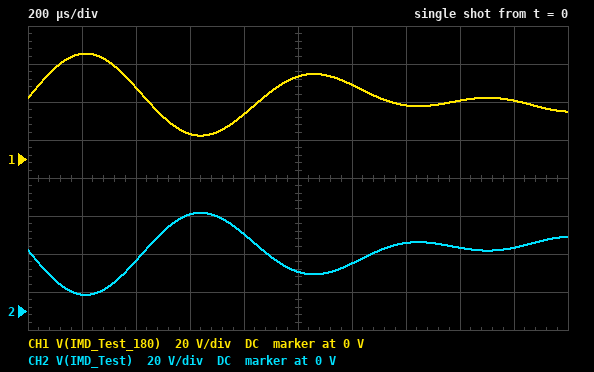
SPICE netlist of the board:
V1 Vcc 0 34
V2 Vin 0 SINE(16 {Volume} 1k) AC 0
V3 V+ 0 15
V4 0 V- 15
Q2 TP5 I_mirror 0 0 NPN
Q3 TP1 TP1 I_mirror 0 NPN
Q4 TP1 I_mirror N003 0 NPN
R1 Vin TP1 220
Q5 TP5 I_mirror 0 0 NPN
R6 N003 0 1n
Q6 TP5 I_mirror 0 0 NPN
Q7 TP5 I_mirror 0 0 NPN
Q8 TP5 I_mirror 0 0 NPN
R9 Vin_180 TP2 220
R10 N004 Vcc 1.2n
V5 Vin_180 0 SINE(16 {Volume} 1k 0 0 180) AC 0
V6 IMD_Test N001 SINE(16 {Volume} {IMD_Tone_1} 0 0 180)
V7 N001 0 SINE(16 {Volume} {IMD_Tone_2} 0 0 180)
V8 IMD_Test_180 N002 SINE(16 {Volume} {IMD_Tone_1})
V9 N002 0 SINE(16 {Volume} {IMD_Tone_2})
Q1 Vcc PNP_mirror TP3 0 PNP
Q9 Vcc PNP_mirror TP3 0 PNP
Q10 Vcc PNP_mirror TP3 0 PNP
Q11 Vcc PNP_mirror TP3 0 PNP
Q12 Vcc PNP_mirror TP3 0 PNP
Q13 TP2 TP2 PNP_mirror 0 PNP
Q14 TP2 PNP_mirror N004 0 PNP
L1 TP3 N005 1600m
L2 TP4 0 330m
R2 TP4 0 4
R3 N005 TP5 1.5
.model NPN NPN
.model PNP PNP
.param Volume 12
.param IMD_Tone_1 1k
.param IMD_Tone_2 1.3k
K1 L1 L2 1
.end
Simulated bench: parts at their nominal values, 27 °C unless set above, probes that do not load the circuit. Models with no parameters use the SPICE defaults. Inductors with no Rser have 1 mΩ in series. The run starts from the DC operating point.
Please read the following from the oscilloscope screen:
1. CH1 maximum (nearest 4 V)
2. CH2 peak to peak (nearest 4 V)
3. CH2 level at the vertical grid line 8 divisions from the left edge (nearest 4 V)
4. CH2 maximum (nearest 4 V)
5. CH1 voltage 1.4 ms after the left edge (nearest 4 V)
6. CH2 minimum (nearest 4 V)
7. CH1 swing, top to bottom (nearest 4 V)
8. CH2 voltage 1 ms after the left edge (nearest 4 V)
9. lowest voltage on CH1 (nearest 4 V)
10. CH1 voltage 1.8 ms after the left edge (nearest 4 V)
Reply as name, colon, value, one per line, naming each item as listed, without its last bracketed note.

CH1 maximum: 56 V
CH2 peak to peak: 44 V
CH2 level at the vertical grid line 8 divisions from the left edge: 32 V
CH2 maximum: 52 V
CH1 voltage 1.4 ms after the left edge: 28 V
CH2 minimum: 8 V
CH1 swing, top to bottom: 44 V
CH2 voltage 1 ms after the left edge: 20 V
lowest voltage on CH1: 12 V
CH1 voltage 1.8 ms after the left edge: 32 V
